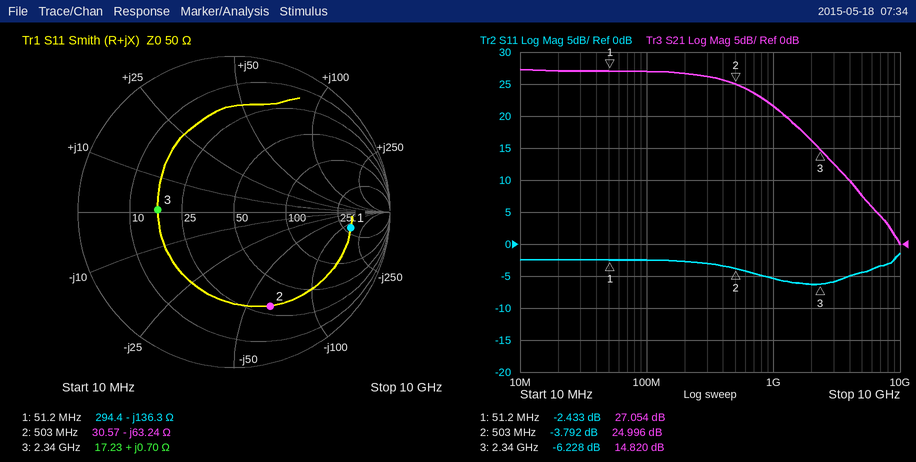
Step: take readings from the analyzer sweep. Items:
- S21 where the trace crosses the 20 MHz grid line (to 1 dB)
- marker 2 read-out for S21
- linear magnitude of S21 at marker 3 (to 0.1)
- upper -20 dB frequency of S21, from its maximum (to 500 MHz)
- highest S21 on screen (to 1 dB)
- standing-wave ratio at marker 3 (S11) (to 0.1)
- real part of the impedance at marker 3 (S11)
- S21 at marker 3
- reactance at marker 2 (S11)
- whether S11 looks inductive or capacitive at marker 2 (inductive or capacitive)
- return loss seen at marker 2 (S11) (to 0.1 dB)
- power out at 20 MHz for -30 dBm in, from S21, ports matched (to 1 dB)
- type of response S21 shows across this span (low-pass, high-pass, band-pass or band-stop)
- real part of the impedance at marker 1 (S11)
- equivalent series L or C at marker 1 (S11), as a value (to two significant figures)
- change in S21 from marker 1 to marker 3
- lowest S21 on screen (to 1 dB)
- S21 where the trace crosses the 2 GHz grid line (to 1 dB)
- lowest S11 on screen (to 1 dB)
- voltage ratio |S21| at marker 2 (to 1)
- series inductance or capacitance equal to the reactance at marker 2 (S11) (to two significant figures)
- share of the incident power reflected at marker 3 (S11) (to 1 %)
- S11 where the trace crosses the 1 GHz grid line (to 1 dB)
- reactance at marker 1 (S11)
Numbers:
27 dB
24.996 dB
5.5
5.0 GHz
27 dB
2.9
17.23 Ω
14.820 dB
-63.24 Ω
capacitive
3.8 dB
-3 dBm
low-pass
294.4 Ω
23 pF
-12.234 dB
0 dB
16 dB
-6 dB
18
5.0 pF
24 %
-5 dB
-136.3 Ω
